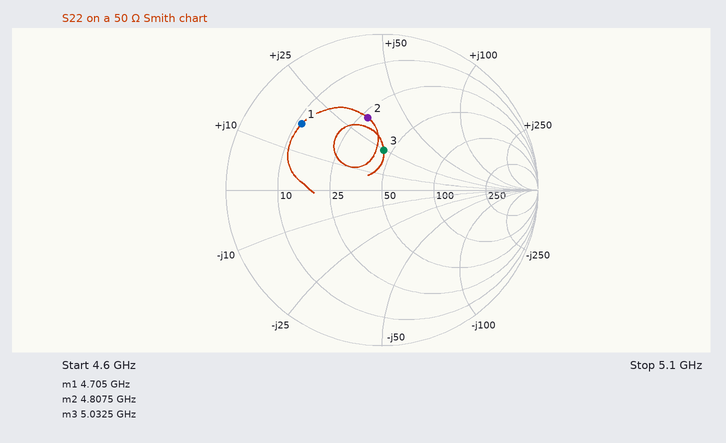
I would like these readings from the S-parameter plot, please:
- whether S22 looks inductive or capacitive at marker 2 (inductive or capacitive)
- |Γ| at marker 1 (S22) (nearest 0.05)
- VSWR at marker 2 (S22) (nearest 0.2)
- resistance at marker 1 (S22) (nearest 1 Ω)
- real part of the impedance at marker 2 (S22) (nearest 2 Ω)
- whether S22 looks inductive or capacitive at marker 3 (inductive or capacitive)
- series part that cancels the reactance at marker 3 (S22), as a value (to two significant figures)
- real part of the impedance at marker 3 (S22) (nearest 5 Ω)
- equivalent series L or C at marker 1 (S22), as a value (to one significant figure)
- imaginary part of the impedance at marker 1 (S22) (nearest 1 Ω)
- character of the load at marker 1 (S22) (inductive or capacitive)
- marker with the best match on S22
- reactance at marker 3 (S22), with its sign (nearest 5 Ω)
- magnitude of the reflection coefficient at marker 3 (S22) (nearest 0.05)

inductive
0.65
2.8
11 Ω
28 Ω
inductive
1.3 pF
45 Ω
600 pH
+17 Ω
inductive
marker 3
+25 Ω
0.25
